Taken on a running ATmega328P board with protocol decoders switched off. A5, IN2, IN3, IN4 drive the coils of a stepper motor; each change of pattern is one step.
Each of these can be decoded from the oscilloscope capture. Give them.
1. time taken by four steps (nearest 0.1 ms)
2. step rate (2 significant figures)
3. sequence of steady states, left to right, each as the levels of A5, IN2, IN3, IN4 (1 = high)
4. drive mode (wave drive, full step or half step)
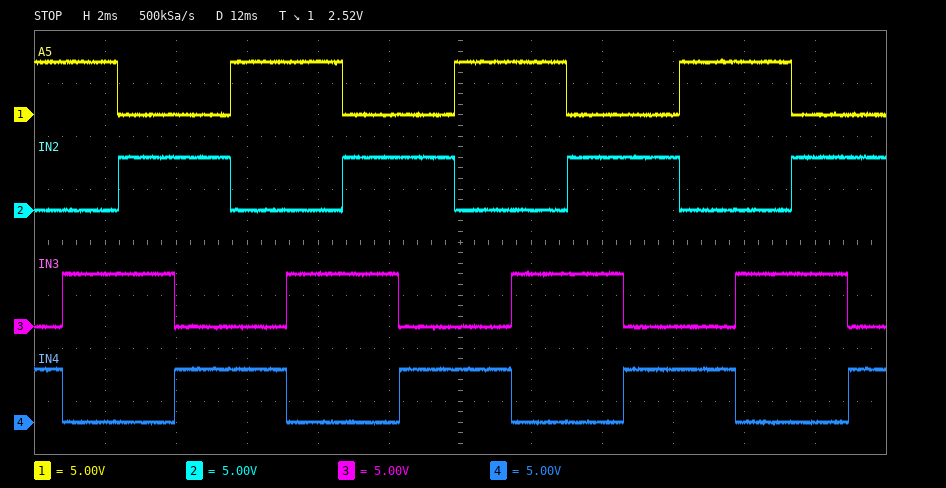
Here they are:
6.3 ms
630 steps/s
1001 1010 0110 0101 1001 1010 0110 0101 1001 1010 0110 0101 1001 1010 0110 0101
full step
